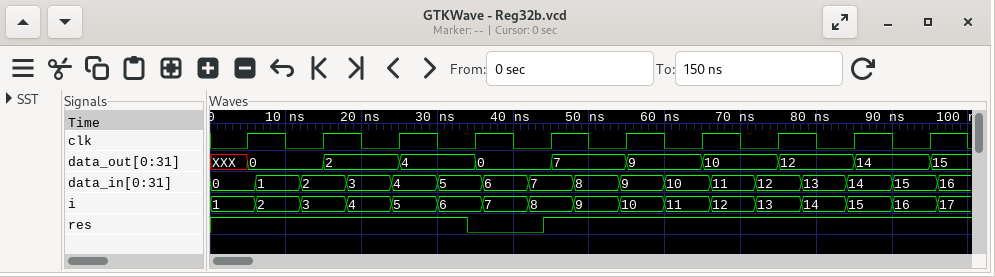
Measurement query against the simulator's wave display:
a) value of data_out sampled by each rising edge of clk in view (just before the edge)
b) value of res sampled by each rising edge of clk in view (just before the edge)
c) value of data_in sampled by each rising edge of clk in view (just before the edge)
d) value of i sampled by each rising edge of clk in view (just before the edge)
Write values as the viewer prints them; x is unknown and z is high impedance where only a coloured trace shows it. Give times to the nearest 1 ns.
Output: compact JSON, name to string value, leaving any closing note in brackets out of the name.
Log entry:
{"value of data_out sampled by each rising edge of clk in view": "XXX, 0, 2, 4, 0, 7, 9, 10, 12, 14", "value of res sampled by each rising edge of clk in view": "1 1 1 0 1 1 1 1 1 1", "value of data_in sampled by each rising edge of clk in view": "0, 2, 4, 5, 7, 9, 10, 12, 14, 15", "value of i sampled by each rising edge of clk in view": "1, 3, 5, 6, 8, 10, 11, 13, 15, 16"}
